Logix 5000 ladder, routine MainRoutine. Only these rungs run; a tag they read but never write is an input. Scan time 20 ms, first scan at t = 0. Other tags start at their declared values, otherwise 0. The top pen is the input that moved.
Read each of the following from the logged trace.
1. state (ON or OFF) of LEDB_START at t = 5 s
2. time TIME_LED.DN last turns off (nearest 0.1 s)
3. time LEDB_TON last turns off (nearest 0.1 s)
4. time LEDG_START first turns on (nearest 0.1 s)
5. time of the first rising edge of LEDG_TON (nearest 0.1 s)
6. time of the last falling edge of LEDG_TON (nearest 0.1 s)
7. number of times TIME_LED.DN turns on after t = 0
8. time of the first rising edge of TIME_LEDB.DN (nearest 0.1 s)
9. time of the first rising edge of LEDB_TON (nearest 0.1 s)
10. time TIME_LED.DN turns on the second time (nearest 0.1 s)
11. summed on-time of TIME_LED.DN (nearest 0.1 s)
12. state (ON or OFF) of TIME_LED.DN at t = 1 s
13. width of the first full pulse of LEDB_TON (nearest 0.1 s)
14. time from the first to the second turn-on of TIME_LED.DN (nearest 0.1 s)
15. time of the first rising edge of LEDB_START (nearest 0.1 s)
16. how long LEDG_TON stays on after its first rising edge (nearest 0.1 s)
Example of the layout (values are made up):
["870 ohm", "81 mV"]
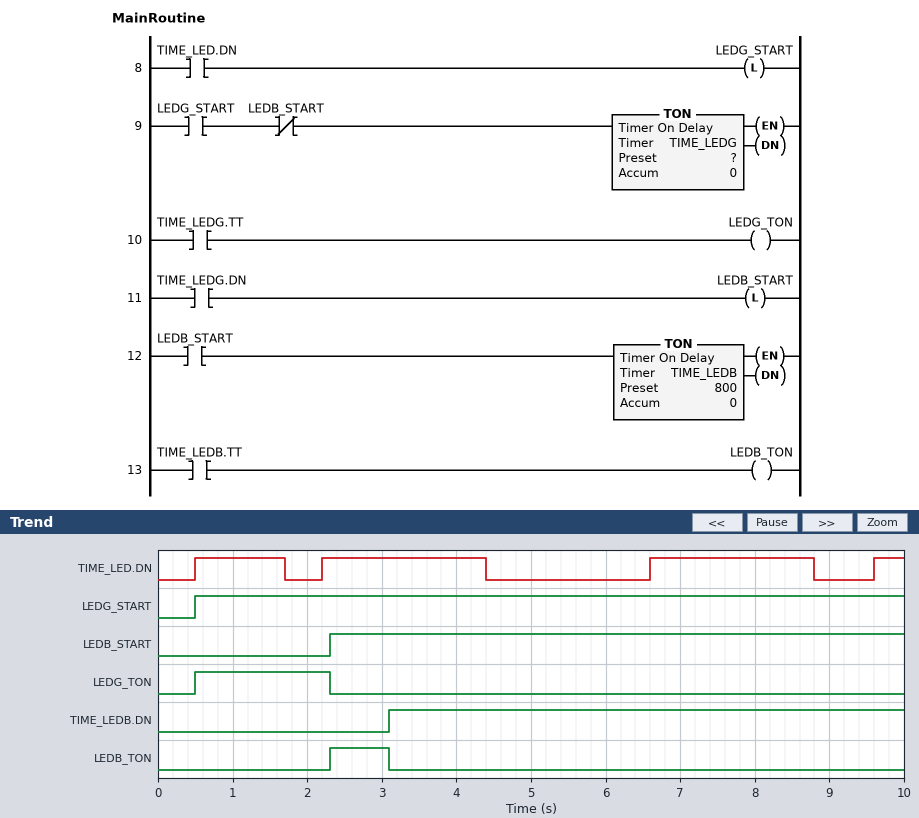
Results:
["ON", "8.8 s", "3.1 s", "0.5 s", "0.5 s", "2.3 s", "4", "3.1 s", "2.3 s", "2.2 s", "6.0 s", "ON", "0.8 s", "1.7 s", "2.3 s", "1.8 s"]
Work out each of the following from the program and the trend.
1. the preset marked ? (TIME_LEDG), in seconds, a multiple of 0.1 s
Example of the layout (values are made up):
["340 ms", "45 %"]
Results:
["1.8 s"]
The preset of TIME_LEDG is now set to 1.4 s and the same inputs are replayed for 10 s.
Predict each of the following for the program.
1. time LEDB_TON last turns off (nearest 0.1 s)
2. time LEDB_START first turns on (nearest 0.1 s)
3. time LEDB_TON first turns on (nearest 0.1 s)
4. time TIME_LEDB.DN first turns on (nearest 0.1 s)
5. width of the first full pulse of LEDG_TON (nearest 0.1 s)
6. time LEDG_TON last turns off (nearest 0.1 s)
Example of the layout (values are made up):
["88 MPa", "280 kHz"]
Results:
["2.7 s", "1.9 s", "1.9 s", "2.7 s", "1.4 s", "1.9 s"]
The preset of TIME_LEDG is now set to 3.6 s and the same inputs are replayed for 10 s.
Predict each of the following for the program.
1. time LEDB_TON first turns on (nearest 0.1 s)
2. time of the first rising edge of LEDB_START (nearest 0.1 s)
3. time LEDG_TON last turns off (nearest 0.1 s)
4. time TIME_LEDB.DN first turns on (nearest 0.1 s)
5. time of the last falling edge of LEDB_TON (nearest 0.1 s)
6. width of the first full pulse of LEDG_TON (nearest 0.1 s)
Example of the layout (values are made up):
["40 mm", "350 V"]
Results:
["4.1 s", "4.1 s", "4.1 s", "4.9 s", "4.9 s", "3.6 s"]
